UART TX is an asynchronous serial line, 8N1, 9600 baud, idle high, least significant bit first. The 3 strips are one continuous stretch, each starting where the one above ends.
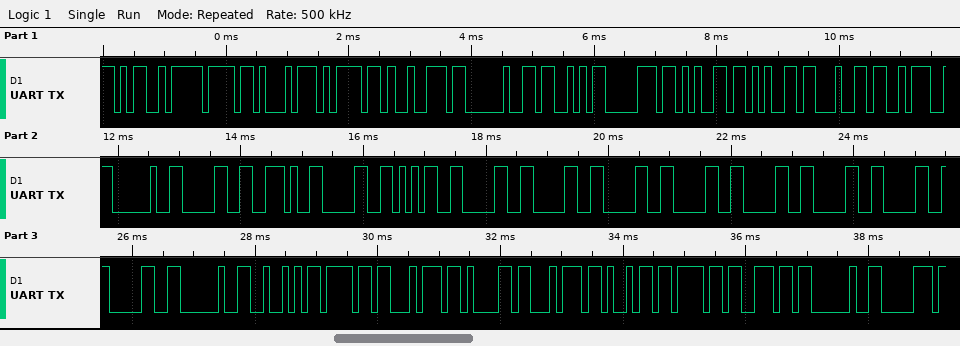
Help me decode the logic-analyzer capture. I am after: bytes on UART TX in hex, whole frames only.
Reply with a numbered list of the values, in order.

1. 4D 6F 74 6F 72 20 53 70 65 65 64 3A 20 30 2E 30 35 30 30 30 30 30 30 30 30 20 52 6F 74 61 74 69 6F 6E 20 70
